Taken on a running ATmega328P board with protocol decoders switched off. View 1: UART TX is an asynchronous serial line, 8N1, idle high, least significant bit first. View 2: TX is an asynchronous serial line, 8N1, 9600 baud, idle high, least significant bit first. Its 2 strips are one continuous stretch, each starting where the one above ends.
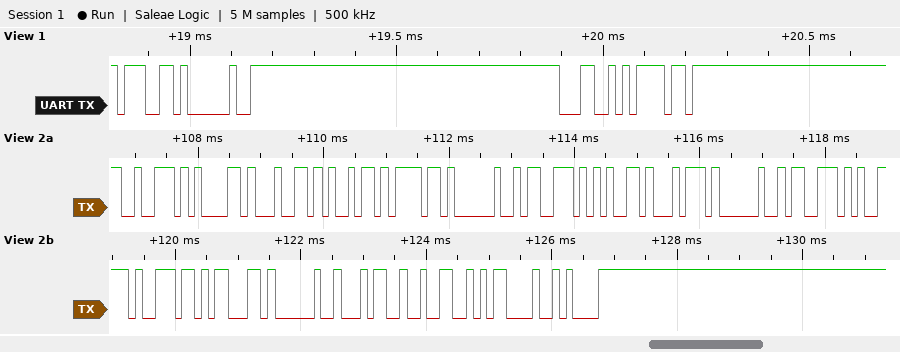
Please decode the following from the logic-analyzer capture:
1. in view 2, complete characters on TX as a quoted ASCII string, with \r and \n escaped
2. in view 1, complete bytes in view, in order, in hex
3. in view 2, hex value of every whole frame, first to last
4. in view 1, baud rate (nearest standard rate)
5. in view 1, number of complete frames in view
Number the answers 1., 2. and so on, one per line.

1. "radio set sync 42\r\n"
2. 0x67 0x20 0x4C 0x6F
3. 0x72 0x61 0x64 0x69 0x6F 0x20 0x73 0x65 0x74 0x20 0x73 0x79 0x6E 0x63 0x20 0x34 0x32 0x0D 0x0A
4. 57600 baud
5. 4
